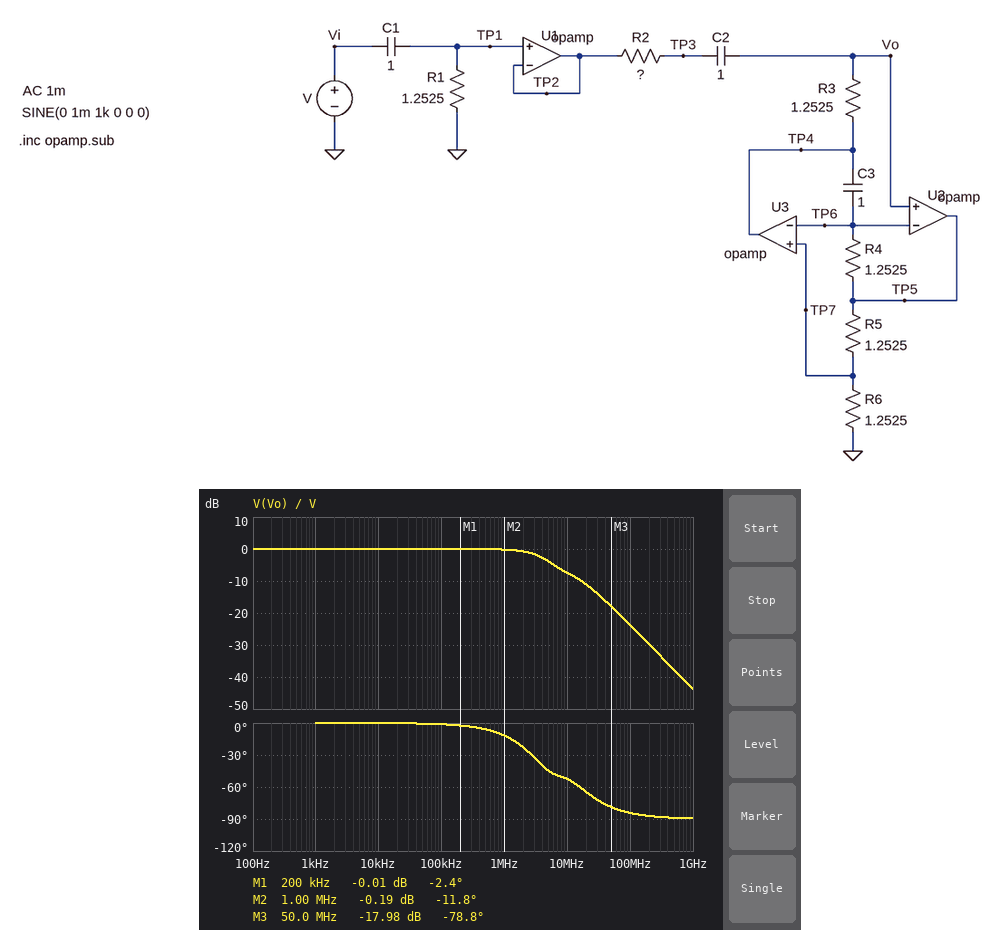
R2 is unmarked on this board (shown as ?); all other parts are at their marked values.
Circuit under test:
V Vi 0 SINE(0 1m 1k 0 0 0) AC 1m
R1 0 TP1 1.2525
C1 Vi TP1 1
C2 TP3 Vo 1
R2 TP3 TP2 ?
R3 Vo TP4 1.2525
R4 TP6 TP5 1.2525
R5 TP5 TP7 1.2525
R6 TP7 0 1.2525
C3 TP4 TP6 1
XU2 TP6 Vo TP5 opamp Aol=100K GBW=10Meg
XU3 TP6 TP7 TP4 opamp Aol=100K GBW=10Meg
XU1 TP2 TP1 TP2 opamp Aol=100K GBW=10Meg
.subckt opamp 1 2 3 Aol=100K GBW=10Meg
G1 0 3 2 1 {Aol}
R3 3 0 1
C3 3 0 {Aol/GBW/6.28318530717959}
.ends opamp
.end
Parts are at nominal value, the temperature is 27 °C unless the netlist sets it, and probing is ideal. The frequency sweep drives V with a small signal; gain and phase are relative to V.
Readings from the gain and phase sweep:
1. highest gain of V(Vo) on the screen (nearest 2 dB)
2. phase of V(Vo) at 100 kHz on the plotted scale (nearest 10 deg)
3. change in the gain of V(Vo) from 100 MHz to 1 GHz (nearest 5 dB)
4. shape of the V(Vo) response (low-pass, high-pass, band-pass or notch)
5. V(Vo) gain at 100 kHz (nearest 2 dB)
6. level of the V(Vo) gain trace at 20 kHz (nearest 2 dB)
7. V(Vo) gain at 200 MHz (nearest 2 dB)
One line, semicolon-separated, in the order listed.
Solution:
0 dB; 0 deg; -20 dB; low-pass; 0 dB; 0 dB; -30 dB
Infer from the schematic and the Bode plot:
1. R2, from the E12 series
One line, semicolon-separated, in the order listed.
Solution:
0.68 Ω
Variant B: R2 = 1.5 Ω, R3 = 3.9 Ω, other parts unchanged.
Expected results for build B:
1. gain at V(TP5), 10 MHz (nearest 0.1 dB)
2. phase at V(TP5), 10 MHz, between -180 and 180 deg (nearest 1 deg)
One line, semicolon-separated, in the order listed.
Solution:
-4.3 dB; -123 deg
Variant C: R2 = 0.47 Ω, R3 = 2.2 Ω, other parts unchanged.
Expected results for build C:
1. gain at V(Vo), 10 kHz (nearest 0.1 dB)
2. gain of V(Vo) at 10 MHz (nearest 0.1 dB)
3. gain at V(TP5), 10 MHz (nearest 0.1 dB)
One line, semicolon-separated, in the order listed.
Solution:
0 dB; -5.0 dB; -3.0 dB
